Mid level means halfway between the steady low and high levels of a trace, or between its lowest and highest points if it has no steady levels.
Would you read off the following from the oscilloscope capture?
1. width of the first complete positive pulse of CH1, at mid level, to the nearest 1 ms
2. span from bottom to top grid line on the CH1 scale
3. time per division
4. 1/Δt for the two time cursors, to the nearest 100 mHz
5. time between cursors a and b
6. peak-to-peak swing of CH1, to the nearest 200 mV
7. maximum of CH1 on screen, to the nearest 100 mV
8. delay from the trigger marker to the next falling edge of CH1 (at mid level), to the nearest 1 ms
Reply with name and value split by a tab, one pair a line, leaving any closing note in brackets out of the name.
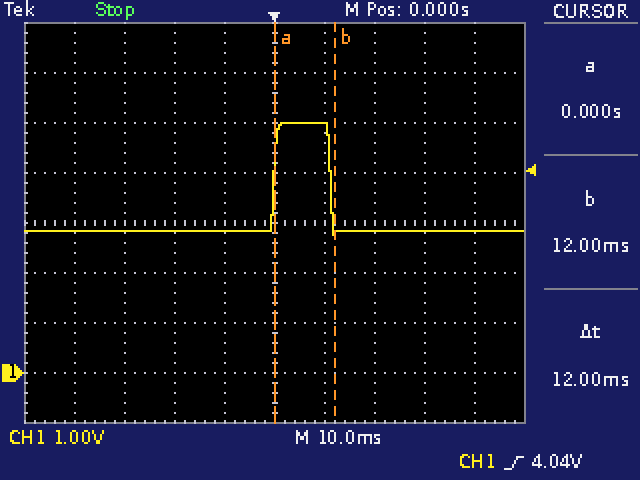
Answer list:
width of the first complete positive pulse of CH1, at mid level, to the nearest 1 ms	11 ms
span from bottom to top grid line on the CH1 scale	8 V
time per division	10 ms
1/Δt for the two time cursors, to the nearest 100 mHz	83.3 Hz
time between cursors a and b	12 ms
peak-to-peak swing of CH1, to the nearest 200 mV	2.2 V
maximum of CH1 on screen, to the nearest 100 mV	5.0 V
delay from the trigger marker to the next falling edge of CH1 (at mid level), to the nearest 1 ms	11 ms
